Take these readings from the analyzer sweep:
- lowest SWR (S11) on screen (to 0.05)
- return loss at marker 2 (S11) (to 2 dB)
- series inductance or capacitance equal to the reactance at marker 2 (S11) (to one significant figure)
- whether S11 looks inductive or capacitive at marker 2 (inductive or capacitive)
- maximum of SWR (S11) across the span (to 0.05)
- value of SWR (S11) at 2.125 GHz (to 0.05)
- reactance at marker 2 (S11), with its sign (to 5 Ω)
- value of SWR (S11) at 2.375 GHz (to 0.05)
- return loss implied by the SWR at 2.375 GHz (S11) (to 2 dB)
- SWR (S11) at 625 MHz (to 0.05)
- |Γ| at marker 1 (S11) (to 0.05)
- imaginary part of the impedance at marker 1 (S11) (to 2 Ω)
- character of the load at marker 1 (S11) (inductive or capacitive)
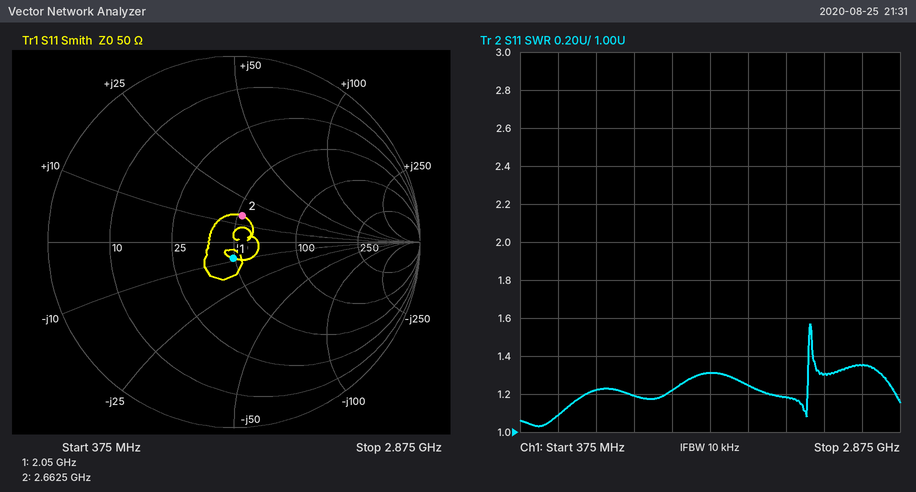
1.05
16 dB
900 pH
inductive
1.55
1.20
+15 Ω
1.30
18 dB
1.10
0.10
-8 Ω
capacitive
